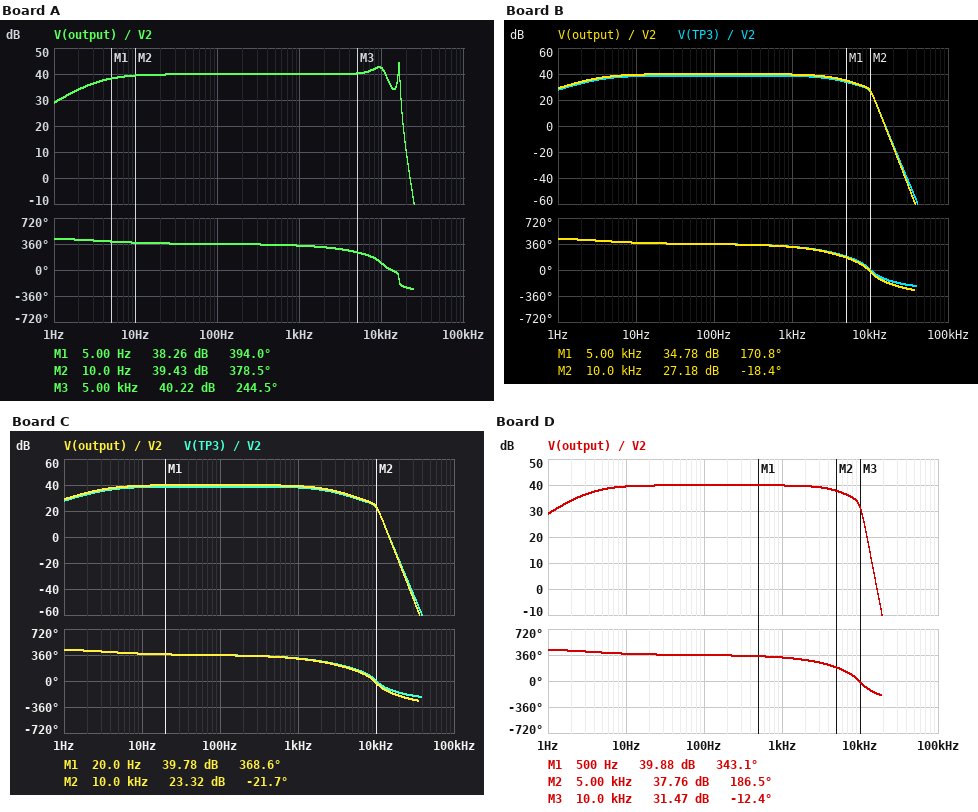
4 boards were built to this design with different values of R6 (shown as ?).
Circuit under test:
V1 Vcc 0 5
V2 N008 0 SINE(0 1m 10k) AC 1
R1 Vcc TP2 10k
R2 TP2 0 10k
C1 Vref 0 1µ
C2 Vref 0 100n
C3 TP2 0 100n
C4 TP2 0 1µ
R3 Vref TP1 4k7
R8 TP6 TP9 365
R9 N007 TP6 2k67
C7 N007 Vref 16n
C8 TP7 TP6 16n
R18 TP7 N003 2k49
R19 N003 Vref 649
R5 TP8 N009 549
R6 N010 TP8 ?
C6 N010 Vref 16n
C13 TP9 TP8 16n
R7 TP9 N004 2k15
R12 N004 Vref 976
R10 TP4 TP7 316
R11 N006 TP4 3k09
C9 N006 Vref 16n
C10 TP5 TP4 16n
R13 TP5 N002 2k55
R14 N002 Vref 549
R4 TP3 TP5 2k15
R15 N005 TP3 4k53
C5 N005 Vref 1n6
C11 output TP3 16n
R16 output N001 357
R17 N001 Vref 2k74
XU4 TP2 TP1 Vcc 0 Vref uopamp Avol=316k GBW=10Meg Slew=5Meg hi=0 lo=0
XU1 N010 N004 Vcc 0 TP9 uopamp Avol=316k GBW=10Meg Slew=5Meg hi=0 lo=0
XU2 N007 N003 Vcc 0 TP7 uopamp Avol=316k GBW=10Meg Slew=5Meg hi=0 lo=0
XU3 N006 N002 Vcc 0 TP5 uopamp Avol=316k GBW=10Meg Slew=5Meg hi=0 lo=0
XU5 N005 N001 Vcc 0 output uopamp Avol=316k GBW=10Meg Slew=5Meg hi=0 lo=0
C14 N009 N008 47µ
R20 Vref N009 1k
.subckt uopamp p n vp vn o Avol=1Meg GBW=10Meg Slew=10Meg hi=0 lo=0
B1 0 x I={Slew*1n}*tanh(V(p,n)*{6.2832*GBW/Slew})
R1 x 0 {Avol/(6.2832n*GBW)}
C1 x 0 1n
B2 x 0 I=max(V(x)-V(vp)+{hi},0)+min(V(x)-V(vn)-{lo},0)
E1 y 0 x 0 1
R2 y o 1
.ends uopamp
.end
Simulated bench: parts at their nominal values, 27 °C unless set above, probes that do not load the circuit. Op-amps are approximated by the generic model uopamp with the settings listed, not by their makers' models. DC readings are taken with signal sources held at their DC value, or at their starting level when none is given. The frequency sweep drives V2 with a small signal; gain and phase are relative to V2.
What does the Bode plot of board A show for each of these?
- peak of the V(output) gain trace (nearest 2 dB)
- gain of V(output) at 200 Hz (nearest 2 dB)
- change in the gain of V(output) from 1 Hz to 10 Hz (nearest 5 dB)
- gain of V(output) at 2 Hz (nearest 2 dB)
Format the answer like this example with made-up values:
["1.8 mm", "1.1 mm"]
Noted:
["44 dB", "40 dB", "10 dB", "34 dB"]
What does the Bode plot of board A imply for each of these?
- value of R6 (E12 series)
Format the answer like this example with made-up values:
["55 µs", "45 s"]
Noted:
["680 Ω"]
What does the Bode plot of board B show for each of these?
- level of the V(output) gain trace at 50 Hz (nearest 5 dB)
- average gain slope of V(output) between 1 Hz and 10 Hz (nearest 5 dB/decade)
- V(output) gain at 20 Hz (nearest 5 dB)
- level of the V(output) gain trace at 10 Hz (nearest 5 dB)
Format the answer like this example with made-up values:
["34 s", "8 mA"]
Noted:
["40 dB", "10 dB/decade", "40 dB", "40 dB"]
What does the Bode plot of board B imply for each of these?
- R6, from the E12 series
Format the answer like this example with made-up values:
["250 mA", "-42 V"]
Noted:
["3.9 kΩ"]
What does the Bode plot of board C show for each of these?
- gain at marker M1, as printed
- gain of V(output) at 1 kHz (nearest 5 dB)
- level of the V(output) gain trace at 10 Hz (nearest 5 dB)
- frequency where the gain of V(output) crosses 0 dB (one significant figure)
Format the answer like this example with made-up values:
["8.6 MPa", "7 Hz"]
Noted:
["39.78 dB", "40 dB", "40 dB", "10 kHz"]
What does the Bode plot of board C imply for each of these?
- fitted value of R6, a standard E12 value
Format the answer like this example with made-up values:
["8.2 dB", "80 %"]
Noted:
["5.6 kΩ"]
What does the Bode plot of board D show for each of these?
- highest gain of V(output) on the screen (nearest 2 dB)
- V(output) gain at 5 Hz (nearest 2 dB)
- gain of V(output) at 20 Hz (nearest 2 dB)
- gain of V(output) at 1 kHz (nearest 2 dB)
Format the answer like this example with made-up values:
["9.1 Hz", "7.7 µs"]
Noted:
["40 dB", "38 dB", "40 dB", "40 dB"]
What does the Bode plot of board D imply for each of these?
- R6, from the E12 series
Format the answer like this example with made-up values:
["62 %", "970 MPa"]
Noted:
["2.7 kΩ"]
